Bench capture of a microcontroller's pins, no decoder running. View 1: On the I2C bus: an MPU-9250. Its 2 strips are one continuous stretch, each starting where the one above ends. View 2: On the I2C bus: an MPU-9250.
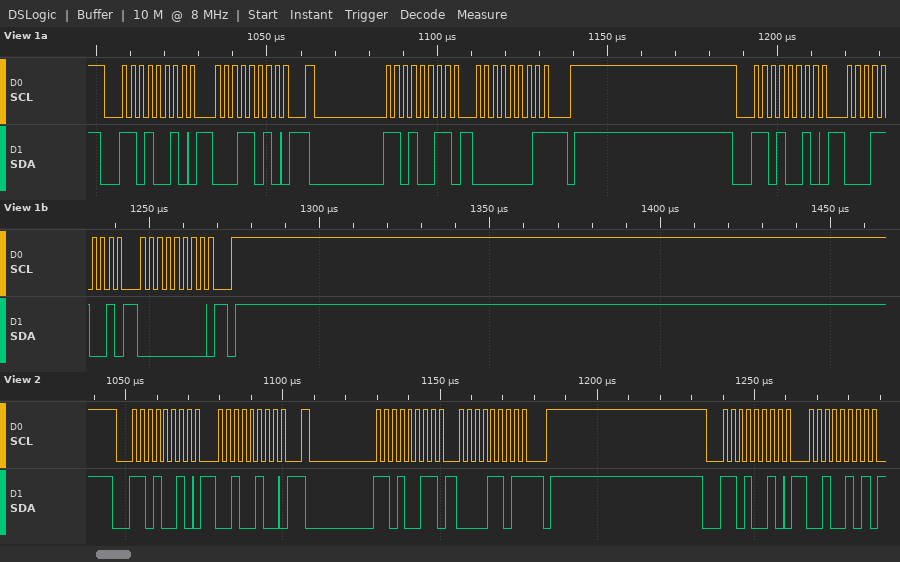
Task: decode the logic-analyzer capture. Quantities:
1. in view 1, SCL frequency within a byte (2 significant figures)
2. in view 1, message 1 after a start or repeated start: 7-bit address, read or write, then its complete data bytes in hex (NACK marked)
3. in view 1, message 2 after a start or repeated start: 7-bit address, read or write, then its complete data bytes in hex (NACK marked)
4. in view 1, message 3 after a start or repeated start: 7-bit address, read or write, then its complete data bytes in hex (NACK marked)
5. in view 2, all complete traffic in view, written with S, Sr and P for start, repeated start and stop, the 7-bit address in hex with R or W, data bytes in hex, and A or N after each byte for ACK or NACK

400 kHz
0x69 write: 1A
0x69 read: 01 NACK
0x69 write: 19 00
S 69W A 24 A Sr 69R A 0D N P S 69W A 25 A
